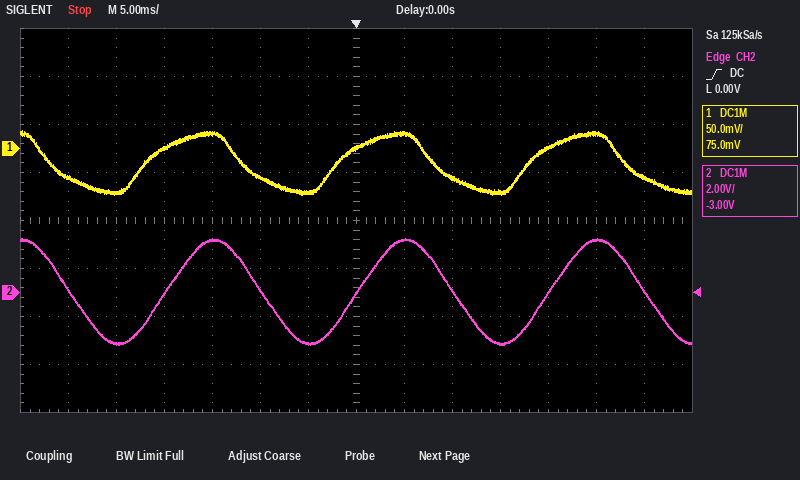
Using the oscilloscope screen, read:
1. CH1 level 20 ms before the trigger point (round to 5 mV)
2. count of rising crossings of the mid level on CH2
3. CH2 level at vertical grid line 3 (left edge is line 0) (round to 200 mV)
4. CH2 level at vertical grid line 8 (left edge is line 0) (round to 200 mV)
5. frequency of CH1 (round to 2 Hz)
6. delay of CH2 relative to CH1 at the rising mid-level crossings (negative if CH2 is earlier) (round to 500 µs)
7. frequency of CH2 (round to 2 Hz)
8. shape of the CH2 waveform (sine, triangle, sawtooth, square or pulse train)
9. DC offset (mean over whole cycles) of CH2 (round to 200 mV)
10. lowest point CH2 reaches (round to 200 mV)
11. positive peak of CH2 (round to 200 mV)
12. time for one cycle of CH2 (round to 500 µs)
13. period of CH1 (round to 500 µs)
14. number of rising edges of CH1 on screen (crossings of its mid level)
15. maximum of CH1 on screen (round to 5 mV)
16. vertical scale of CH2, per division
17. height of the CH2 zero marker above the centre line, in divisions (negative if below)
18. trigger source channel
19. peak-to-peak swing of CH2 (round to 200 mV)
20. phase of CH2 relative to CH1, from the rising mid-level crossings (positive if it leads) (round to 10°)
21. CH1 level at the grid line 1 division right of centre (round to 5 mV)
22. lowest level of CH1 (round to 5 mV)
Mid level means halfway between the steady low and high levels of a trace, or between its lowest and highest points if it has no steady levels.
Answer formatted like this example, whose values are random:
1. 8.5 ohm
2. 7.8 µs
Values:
1. 0 mV
2. 3
3. 0.0 V
4. 2.2 V
5. 50 Hz
6. +2.0 ms
7. 50 Hz
8. sine
9. 0.0 V
10. -2.2 V
11. 2.2 V
12. 20.0 ms
13. 20.0 ms
14. 3
15. 20 mV
16. 2 V
17. -1.5 div
18. CH2
19. 4.4 V
20. -40°
21. 15 mV
22. -50 mV
